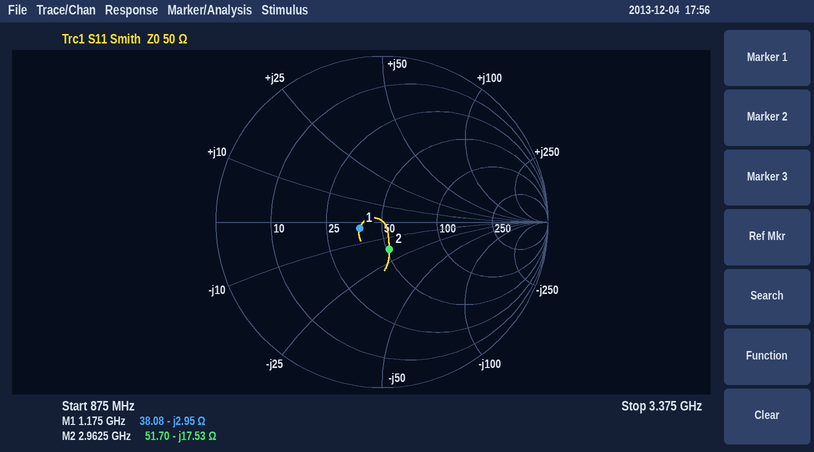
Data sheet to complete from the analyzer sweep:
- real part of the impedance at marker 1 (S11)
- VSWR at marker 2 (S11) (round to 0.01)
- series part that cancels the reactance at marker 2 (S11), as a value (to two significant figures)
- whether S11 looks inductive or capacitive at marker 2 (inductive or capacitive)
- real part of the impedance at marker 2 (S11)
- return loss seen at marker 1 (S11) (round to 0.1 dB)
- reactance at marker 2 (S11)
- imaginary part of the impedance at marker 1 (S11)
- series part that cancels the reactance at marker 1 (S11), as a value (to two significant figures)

38.08 Ω
1.41
940 pH
capacitive
51.70 Ω
17.1 dB
-17.53 Ω
-2.95 Ω
400 pH
